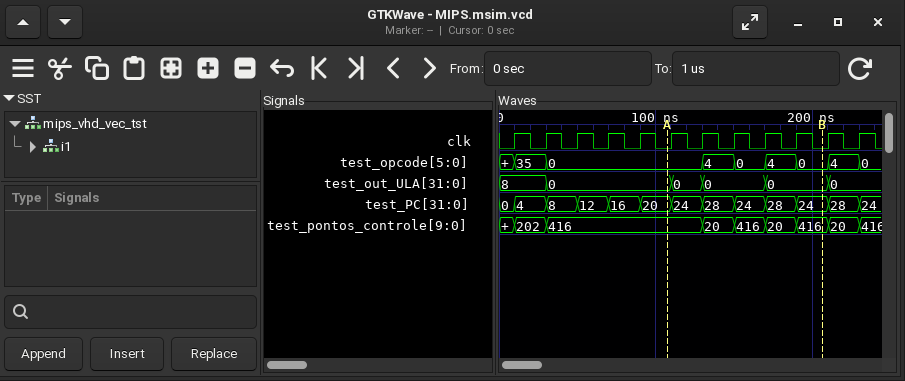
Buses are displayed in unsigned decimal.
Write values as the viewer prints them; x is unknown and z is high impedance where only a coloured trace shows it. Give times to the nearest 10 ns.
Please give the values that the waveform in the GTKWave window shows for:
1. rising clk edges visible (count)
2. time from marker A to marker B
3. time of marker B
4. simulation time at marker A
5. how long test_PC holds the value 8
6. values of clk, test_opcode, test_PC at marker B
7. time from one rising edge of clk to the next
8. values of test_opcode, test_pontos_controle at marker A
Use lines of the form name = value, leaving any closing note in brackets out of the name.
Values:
rising clk edges visible = 12
time from marker A to marker B = 100 ns
time of marker B = 210 ns
simulation time at marker A = 110 ns
how long test_PC holds the value 8 = 20 ns
values of clk, test_opcode, test_PC at marker B = clk=0, test_opcode=0, test_PC=24
time from one rising edge of clk to the next = 20 ns
values of test_opcode, test_pontos_controle at marker A = test_opcode=0, test_pontos_controle=416
